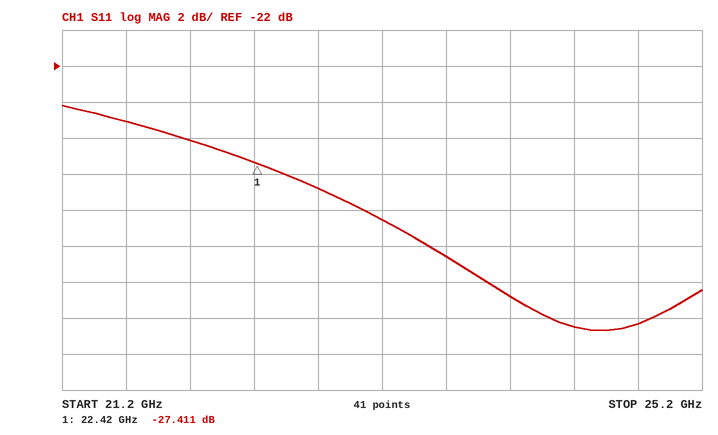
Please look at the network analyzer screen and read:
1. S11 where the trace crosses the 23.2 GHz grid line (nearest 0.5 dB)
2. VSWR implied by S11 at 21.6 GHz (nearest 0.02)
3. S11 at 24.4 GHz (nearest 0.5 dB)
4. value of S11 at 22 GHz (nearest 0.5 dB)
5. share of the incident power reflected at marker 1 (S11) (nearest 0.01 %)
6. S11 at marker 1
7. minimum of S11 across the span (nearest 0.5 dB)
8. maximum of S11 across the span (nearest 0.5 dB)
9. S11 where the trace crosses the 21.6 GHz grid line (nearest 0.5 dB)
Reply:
-30.5 dB
1.12
-36.5 dB
-26.0 dB
0.18 %
-27.411 dB
-36.5 dB
-24.0 dB
-25.0 dB
